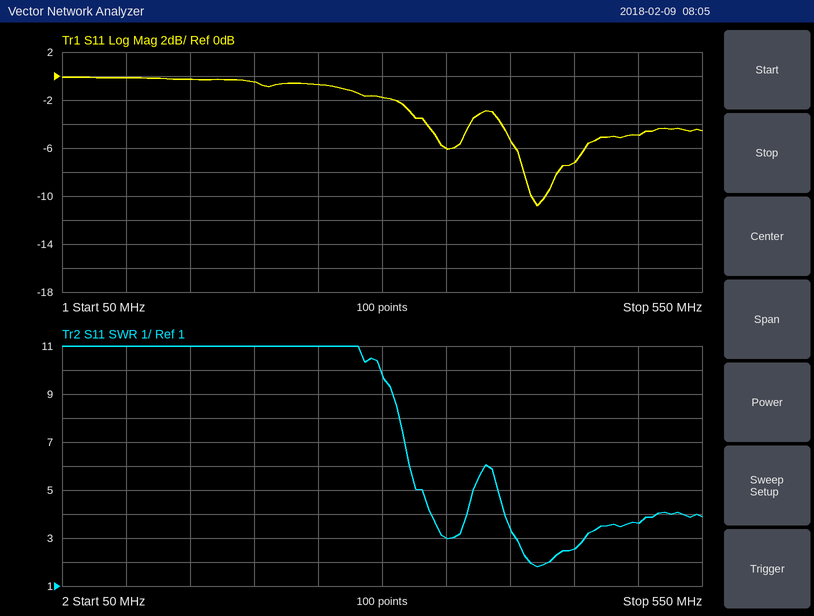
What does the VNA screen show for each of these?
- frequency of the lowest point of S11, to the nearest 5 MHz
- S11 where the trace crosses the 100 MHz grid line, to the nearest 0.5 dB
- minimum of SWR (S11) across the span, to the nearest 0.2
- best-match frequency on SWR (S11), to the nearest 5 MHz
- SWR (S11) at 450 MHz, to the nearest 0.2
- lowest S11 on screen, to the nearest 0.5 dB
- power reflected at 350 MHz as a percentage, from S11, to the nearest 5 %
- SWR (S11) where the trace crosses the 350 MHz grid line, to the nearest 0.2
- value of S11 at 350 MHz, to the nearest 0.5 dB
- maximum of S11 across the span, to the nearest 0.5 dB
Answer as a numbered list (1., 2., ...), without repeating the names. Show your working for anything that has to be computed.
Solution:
1. 420 MHz
2. 0.0 dB
3. 1.8
4. 420 MHz
5. 2.6
6. -11.0 dB
7. 10^(-6/10) ≈ 25 %
8. 3.0
9. -6.0 dB
10. 0.0 dB
